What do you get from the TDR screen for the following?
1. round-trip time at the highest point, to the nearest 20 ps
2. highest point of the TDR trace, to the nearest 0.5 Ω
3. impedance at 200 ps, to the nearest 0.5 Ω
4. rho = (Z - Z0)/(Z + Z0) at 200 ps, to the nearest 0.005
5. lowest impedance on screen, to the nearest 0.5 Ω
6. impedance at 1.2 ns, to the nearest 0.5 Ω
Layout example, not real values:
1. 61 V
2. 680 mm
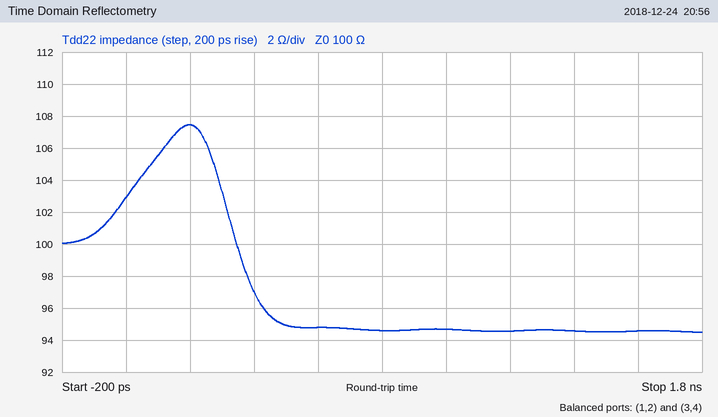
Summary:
1. 200 ps
2. 107.5 Ω
3. 107.5 Ω
4. +0.035
5. 94.5 Ω
6. 94.5 Ω
